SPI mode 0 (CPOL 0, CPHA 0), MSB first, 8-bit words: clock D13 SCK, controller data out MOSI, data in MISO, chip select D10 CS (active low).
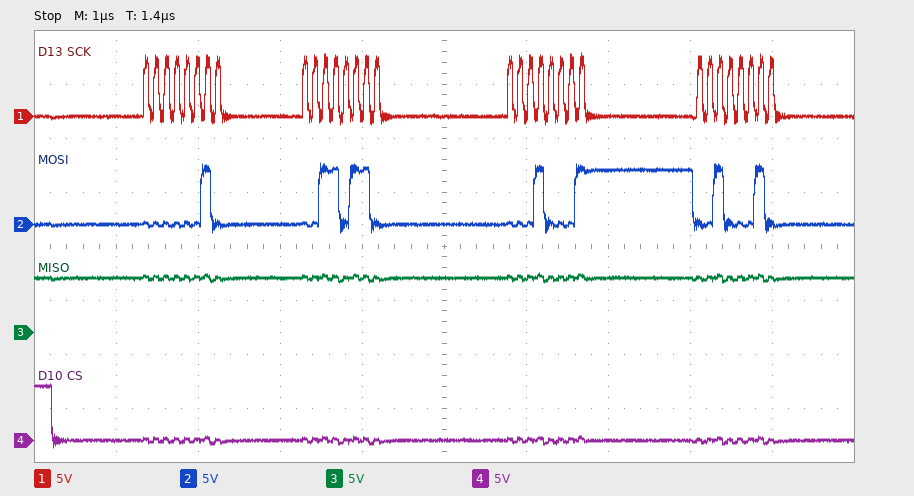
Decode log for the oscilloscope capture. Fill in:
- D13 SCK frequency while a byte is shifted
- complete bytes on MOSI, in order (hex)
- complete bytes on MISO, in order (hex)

8 MHz
02 36 11 22
FF FF FF FF
